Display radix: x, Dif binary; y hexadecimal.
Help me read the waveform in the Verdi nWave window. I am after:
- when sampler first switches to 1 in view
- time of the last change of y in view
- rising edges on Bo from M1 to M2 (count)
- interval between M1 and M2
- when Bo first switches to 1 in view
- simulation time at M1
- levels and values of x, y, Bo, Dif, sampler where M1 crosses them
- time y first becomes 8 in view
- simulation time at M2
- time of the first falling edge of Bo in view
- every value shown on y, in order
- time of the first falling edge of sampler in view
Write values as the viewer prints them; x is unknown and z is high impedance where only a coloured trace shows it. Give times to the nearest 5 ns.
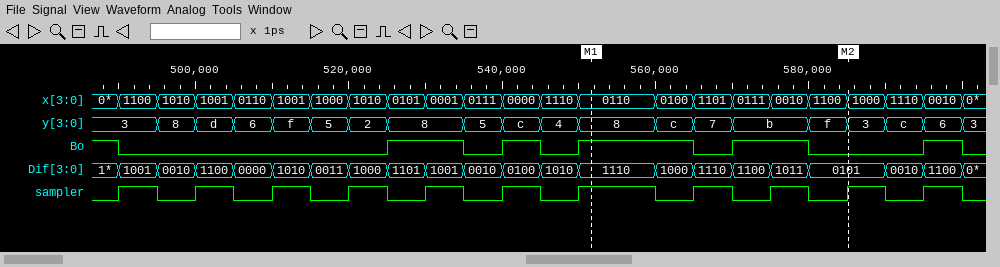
490 ns
600 ns
1
35 ns
525 ns
550 ns
x=0110, y=8, Bo=1, Dif=1110, sampler=1
495 ns
585 ns
490 ns
3, 8, d, 6, f, 5, 2, 8, 5, c, 4, 8, c, 7, b, f, 3, c, 6, 3
495 ns
